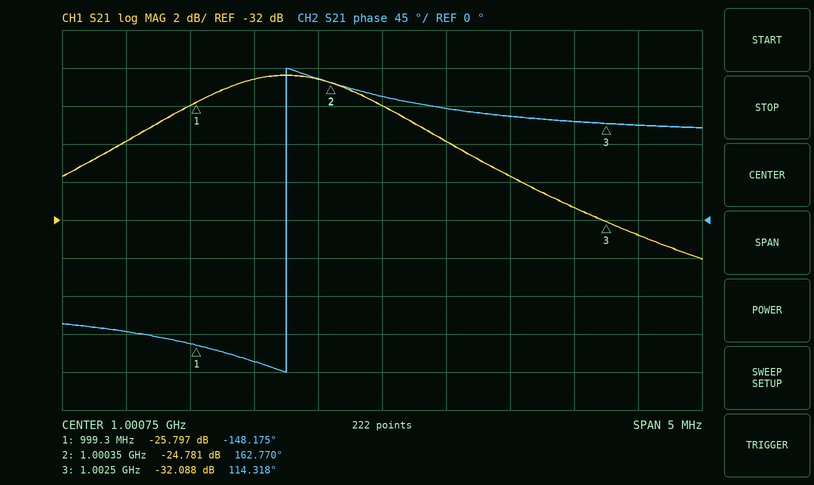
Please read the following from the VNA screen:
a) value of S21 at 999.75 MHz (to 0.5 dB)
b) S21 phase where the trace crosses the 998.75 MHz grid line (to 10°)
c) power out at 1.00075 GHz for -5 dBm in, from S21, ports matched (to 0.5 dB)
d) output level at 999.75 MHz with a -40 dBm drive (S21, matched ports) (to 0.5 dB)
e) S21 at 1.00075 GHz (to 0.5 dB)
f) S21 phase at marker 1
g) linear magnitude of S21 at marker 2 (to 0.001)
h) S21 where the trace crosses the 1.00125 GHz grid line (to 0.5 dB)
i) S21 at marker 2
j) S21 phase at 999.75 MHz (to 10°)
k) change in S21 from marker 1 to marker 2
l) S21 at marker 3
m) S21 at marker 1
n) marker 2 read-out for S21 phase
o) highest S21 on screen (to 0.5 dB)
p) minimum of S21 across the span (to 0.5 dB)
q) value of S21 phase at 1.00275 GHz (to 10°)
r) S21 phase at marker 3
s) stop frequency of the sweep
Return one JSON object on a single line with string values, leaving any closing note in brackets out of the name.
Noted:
{"value of S21 at 999.75 MHz": "-24.5 dB", "S21 phase where the trace crosses the 998.75 MHz grid line": "-130°", "power out at 1.00075 GHz for -5 dBm in, from S21, ports matched": "-31.0 dBm", "output level at 999.75 MHz with a -40 dBm drive (S21, matched ports)": "-64.5 dBm", "S21 at 1.00075 GHz": "-26.0 dB", "S21 phase at marker 1": "-148.175°", "linear magnitude of S21 at marker 2": "0.058", "S21 where the trace crosses the 1.00125 GHz grid line": "-28.0 dB", "S21 at marker 2": "-24.781 dB", "S21 phase at 999.75 MHz": "-170°", "change in S21 from marker 1 to marker 2": "1.016 dB", "S21 at marker 3": "-32.088 dB", "S21 at marker 1": "-25.797 dB", "marker 2 read-out for S21 phase": "162.770°", "highest S21 on screen": "-24.5 dB", "minimum of S21 across the span": "-34.0 dB", "value of S21 phase at 1.00275 GHz": "110°", "S21 phase at marker 3": "114.318°", "stop frequency of the sweep": "1.00325 GHz"}
